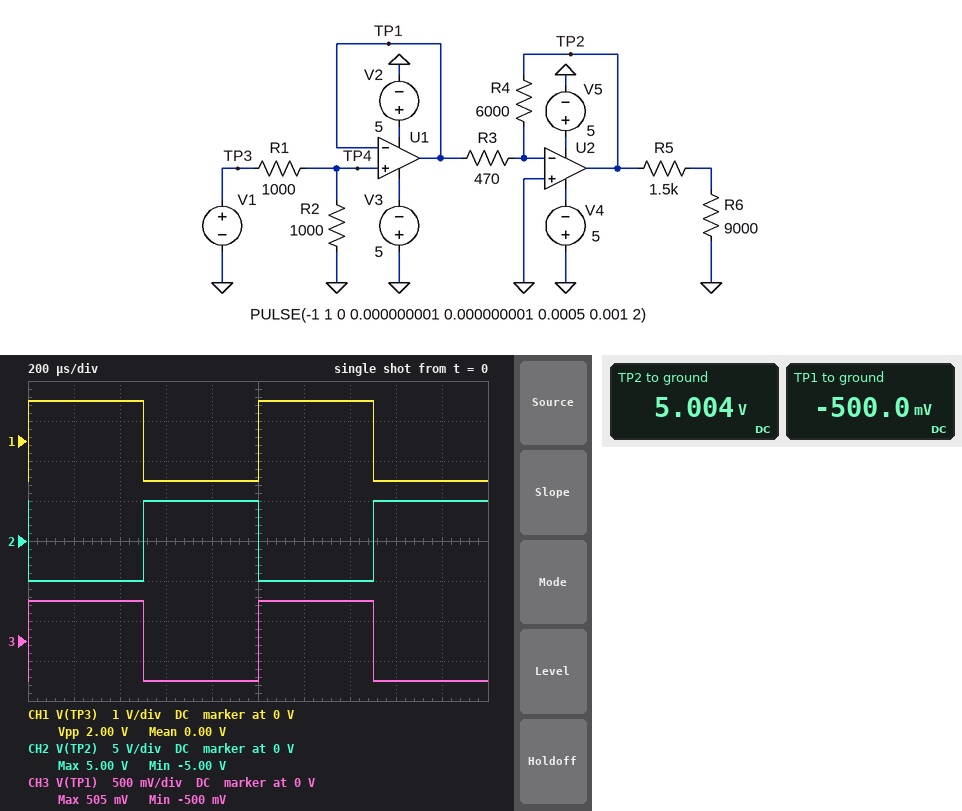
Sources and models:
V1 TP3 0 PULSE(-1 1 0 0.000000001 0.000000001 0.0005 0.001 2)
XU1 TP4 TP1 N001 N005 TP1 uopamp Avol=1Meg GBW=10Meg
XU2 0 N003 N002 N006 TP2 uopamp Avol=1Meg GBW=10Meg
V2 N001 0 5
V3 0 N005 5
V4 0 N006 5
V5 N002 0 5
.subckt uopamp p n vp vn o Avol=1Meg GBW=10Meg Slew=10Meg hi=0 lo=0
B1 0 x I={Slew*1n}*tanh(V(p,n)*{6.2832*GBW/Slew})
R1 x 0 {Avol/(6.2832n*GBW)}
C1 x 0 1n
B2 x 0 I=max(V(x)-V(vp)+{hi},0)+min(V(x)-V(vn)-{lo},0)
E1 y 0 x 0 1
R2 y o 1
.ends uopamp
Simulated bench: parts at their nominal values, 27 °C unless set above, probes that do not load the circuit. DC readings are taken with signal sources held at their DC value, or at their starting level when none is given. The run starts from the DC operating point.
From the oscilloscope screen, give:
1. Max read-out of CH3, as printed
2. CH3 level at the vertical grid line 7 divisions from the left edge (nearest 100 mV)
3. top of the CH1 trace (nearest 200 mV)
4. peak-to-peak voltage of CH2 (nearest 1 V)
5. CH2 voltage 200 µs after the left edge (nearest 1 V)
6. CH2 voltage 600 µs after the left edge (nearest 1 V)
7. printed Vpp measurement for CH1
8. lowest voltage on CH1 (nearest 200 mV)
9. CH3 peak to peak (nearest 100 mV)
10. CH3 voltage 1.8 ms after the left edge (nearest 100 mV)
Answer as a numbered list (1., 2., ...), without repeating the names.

1. 505 mV
2. 500 mV
3. 1.0 V
4. 10 V
5. -5 V
6. 5 V
7. 2.00 V
8. -1.0 V
9. 1.0 V
10. -500 mV
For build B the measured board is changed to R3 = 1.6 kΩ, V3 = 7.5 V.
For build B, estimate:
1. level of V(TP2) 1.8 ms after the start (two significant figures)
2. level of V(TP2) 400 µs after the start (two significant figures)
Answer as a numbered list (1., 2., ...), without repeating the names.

1. 1.9 V
2. -1.9 V
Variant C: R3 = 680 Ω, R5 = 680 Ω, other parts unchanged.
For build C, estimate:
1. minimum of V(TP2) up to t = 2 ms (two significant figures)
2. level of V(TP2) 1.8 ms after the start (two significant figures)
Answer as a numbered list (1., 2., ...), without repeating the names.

1. -4.4 V
2. 4.4 V
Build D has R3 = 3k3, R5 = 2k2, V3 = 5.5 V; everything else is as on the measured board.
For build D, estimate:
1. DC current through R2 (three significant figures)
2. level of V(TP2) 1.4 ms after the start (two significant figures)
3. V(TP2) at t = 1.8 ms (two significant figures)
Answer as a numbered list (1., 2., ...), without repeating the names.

1. 500 µA
2. -910 mV
3. 910 mV
